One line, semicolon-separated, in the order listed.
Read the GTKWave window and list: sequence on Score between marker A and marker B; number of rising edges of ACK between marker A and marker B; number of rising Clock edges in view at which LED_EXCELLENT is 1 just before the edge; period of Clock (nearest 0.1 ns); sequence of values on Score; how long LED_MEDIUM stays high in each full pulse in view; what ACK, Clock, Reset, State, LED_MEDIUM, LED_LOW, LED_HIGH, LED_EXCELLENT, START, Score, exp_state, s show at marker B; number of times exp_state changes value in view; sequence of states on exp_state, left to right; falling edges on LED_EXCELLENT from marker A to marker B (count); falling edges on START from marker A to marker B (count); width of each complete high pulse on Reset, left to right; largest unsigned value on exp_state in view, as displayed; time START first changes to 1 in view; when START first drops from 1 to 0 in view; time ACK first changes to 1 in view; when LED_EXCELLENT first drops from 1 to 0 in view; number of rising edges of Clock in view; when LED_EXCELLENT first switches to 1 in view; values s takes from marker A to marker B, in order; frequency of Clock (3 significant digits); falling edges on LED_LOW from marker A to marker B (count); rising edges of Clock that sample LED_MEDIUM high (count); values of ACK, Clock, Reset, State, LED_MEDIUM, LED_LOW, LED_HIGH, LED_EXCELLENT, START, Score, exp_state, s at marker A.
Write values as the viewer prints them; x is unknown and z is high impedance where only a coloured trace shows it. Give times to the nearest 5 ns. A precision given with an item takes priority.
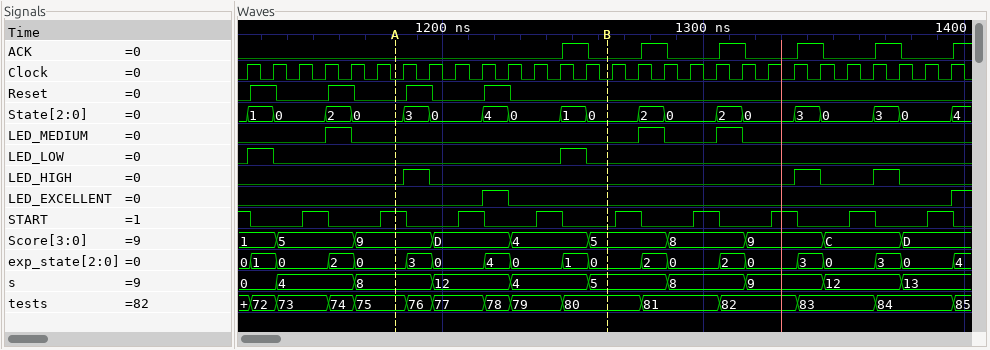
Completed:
9, D, 4, 5; 1; 1; 10 ns; 1, 5, 9, D, 4, 5, 8, 9, C, D; 10 ns, 10 ns, 10 ns; ACK=0, Clock=0, Reset=0, State=0, LED_MEDIUM=0, LED_LOW=0, LED_HIGH=0, LED_EXCELLENT=0, START=0, Score=5, exp_state=0, s=5; 19; 0, 1, 0, 2, 0, 3, 0, 4, 0, 1, 0, 2, 0, 2, 0, 3, 0, 3, 0, 4; 1; 3; 10 ns, 10 ns, 10 ns, 10 ns; 4; 1145 ns; 1125 ns; 1245 ns; 1225 ns; 28; 1215 ns; 8, 12, 4, 5; 100 MHz; 1; 3; ACK=0, Clock=0, Reset=0, State=0, LED_MEDIUM=0, LED_LOW=0, LED_HIGH=0, LED_EXCELLENT=0, START=1, Score=9, exp_state=0, s=8
